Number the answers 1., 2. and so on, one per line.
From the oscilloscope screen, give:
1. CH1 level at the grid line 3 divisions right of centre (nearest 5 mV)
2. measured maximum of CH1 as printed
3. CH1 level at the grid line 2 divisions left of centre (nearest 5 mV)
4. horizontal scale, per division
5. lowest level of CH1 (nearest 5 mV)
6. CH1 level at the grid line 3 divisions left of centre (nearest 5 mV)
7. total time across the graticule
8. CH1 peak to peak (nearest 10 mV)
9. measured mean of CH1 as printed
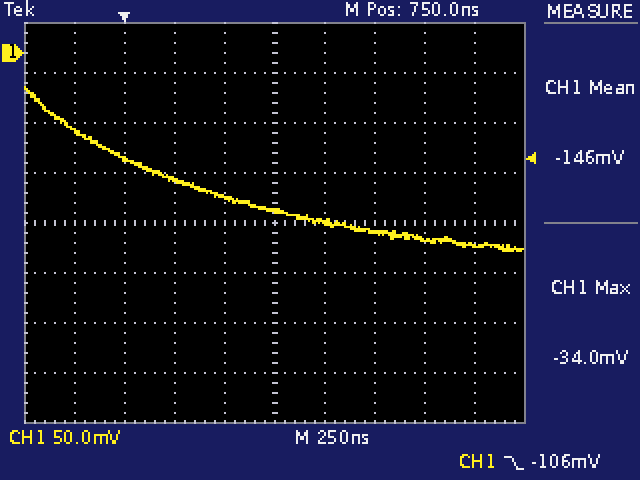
1. -185 mV
2. -34.0 mV
3. -125 mV
4. 250 ns
5. -200 mV
6. -105 mV
7. 2.5 µs
8. 160 mV
9. -146 mV
